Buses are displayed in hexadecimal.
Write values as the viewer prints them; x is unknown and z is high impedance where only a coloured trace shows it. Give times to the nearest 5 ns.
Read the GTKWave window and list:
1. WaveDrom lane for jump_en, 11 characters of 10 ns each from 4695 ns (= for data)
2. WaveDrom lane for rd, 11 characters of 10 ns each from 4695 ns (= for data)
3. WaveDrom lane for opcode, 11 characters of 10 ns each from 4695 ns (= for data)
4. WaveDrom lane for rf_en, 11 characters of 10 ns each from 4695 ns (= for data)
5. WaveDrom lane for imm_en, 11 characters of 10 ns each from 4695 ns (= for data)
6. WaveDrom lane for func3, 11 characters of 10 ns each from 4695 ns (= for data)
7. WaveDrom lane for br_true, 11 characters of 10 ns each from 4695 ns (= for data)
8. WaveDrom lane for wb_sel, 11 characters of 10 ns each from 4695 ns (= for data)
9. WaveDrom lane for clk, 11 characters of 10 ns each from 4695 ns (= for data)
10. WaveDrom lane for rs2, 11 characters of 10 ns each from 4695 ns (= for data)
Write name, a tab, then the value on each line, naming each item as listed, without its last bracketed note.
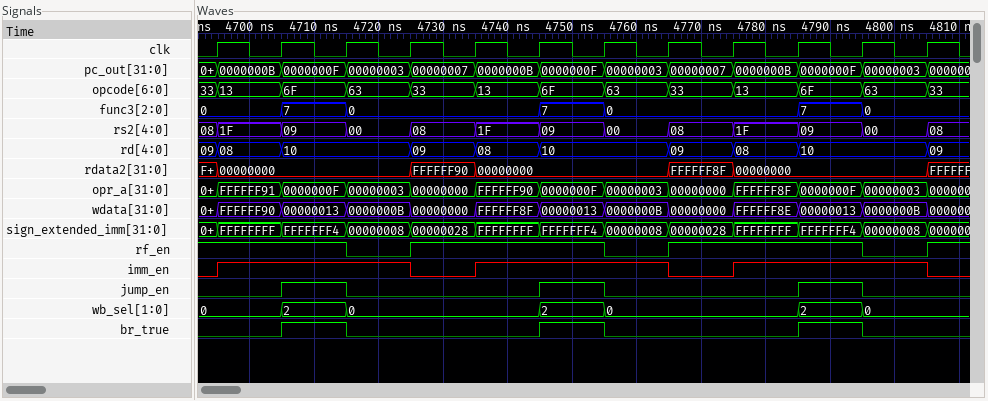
WaveDrom lane for jump_en, 11 characters of 10 ns each from 4695 ns	{name: 'jump_en', wave: '010..10..10'}
WaveDrom lane for rd, 11 characters of 10 ns each from 4695 ns	{name: 'rd', wave: '==.===.===.', data: '08 10 09 08 10 09 08 10'}
WaveDrom lane for opcode, 11 characters of 10 ns each from 4695 ns	{name: 'opcode', wave: '===========', data: '13 6F 63 33 13 6F 63 33 13 6F 63'}
WaveDrom lane for rf_en, 11 characters of 10 ns each from 4695 ns	{name: 'rf_en', wave: '1.01..01..0'}
WaveDrom lane for imm_en, 11 characters of 10 ns each from 4695 ns	{name: 'imm_en', wave: '1..01..01..'}
WaveDrom lane for func3, 11 characters of 10 ns each from 4695 ns	{name: 'func3', wave: '===..==..==', data: '0 7 0 7 0 7 0'}
WaveDrom lane for br_true, 11 characters of 10 ns each from 4695 ns	{name: 'br_true', wave: '010..10..10'}
WaveDrom lane for wb_sel, 11 characters of 10 ns each from 4695 ns	{name: 'wb_sel', wave: '===..==..==', data: '0 2 0 2 0 2 0'}
WaveDrom lane for clk, 11 characters of 10 ns each from 4695 ns	{name: 'clk', wave: 'p..........'}
WaveDrom lane for rs2, 11 characters of 10 ns each from 4695 ns	{name: 'rs2', wave: '===========', data: '1F 09 00 08 1F 09 00 08 1F 09 00'}
